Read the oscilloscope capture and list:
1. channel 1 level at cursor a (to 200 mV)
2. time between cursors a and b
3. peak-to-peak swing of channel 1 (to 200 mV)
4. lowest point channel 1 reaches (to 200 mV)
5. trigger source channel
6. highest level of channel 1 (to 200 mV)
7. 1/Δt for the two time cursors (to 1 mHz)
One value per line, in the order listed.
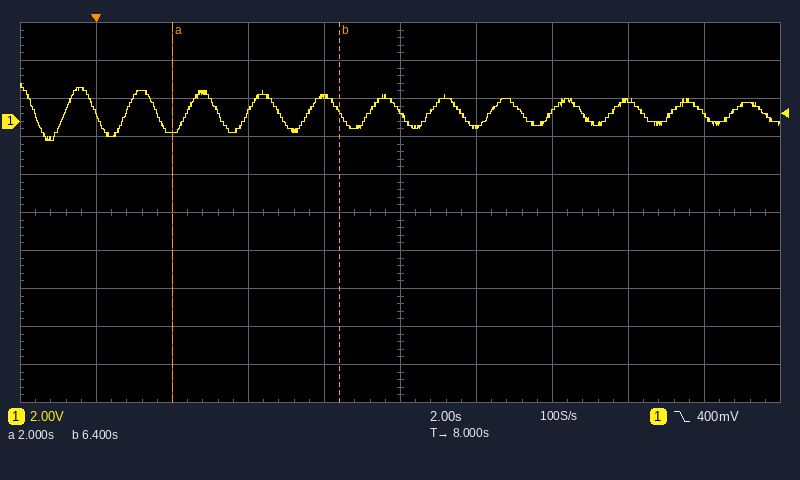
-600 mV
4.4 s
3.0 V
-1.0 V
channel 1
2.0 V
227 mHz
